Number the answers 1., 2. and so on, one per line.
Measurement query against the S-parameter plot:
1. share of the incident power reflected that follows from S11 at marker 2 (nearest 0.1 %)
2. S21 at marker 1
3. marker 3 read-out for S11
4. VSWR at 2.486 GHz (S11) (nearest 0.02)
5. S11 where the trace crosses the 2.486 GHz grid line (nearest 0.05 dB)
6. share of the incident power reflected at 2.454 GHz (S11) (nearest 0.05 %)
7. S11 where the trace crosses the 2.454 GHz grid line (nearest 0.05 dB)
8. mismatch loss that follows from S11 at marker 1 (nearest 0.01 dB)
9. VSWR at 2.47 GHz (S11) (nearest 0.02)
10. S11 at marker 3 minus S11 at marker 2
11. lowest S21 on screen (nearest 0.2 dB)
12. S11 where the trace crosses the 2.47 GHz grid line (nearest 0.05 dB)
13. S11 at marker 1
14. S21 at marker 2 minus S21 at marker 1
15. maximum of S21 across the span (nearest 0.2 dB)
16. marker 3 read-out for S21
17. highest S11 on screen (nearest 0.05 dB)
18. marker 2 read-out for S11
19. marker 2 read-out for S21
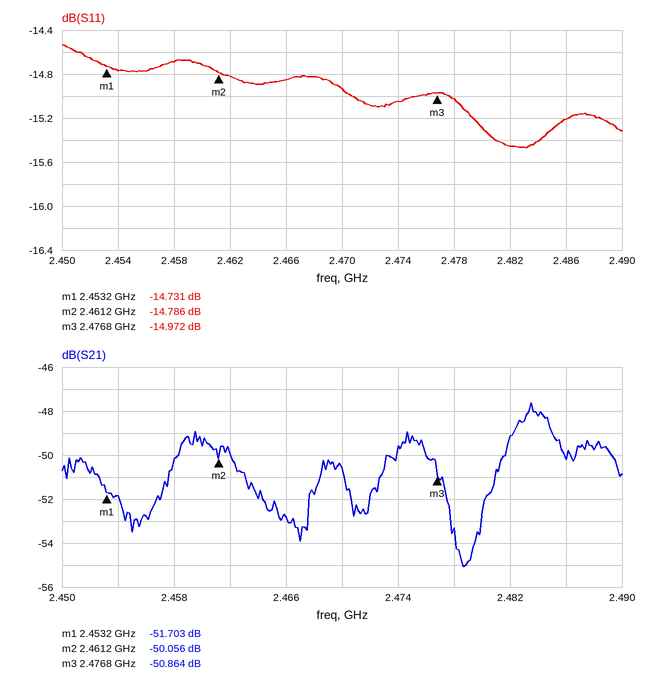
1. 3.3 %
2. -51.703 dB
3. -14.972 dB
4. 1.42
5. -15.20 dB
6. 3.35 %
7. -14.75 dB
8. 0.15 dB
9. 1.44
10. -0.186 dB
11. -55.0 dB
12. -14.95 dB
13. -14.731 dB
14. 1.647 dB
15. -47.6 dB
16. -50.864 dB
17. -14.55 dB
18. -14.786 dB
19. -50.056 dB
